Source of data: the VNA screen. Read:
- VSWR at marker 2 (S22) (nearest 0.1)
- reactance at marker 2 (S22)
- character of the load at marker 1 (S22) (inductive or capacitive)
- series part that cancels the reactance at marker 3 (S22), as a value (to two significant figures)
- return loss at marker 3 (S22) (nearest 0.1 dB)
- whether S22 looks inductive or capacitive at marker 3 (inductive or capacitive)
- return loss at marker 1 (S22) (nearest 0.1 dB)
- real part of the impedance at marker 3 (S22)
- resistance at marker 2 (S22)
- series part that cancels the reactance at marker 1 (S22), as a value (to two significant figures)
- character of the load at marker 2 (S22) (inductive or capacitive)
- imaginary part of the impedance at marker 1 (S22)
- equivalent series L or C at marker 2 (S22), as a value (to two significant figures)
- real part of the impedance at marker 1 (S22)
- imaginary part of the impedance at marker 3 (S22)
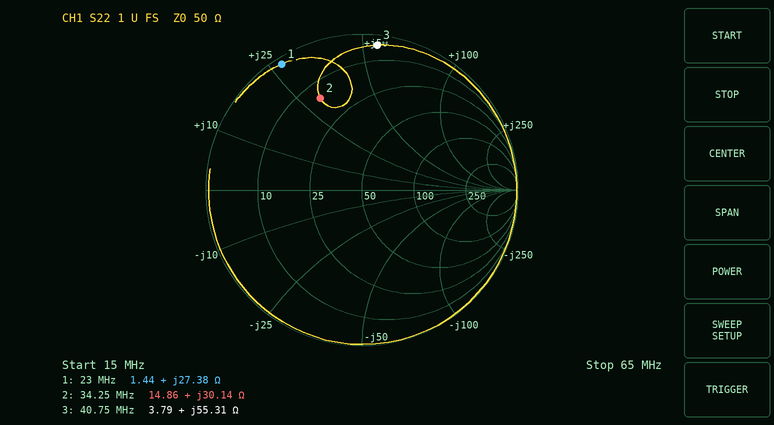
4.7
+30.14 Ω
inductive
71 pF
0.6 dB
inductive
0.4 dB
3.79 Ω
14.86 Ω
250 pF
inductive
+27.38 Ω
140 nH
1.44 Ω
+55.31 Ω
